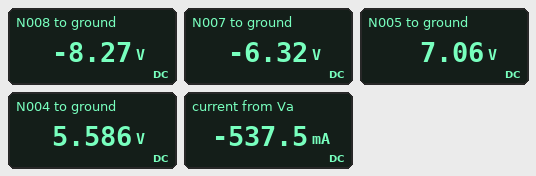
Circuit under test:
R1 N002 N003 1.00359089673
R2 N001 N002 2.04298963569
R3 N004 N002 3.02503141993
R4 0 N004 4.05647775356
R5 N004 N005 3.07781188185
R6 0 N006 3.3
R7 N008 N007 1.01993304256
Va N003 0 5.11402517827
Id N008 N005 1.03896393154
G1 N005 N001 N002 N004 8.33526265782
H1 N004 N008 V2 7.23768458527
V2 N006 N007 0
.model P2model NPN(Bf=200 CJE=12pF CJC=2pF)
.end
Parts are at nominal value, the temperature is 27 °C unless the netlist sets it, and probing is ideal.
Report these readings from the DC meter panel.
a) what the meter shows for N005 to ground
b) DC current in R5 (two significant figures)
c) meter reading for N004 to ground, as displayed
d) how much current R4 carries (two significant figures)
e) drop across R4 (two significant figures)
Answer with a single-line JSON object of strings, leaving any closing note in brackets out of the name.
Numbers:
{"what the meter shows for N005 to ground": "7.06 V", "DC current in R5": "480 mA", "meter reading for N004 to ground, as displayed": "5.586 V", "how much current R4 carries": "1.4 A", "drop across R4": "5.6 V"}
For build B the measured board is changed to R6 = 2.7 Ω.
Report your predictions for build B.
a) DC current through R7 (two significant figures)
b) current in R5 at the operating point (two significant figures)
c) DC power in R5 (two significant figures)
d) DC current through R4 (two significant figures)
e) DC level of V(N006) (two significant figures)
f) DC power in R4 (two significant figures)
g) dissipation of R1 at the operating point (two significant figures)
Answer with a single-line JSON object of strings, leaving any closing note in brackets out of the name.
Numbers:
{"DC current through R7": "1.5 A", "current in R5 at the operating point": "830 mA", "DC power in R5": "2.1 W", "DC current through R4": "1.3 A", "DC level of V(N006)": "-4.1 V", "DC power in R4": "6.9 W", "dissipation of R1 at the operating point": "40 mW"}
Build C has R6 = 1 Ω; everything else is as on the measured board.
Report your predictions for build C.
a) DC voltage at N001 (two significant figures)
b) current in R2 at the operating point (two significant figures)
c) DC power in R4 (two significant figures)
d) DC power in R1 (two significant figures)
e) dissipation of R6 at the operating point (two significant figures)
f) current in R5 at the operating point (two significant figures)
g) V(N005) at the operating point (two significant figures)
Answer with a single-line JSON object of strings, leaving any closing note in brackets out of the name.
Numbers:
{"DC voltage at N001": "4.3 V", "current in R2 at the operating point": "280 mA", "DC power in R4": "5.9 W", "DC power in R1": "72 mW", "dissipation of R6 at the operating point": "870 mW", "current in R5 at the operating point": "1.3 A", "V(N005) at the operating point": "8.9 V"}
